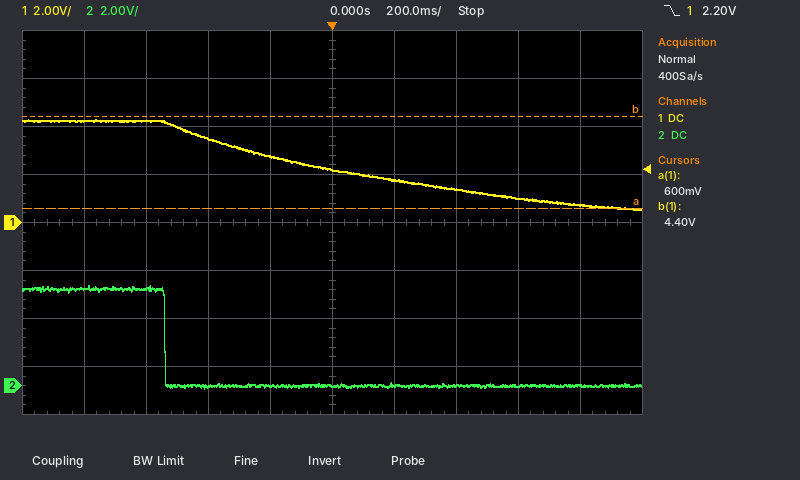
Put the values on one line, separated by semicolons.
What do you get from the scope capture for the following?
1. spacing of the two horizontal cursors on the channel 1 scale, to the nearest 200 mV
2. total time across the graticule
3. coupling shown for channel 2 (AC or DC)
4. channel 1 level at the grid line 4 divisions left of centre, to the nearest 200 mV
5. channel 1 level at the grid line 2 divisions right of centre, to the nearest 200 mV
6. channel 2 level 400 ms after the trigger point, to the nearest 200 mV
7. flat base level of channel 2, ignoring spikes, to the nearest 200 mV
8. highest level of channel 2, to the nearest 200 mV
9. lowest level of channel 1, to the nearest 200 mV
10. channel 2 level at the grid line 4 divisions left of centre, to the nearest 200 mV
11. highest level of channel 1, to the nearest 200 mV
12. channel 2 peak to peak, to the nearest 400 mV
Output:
3.8 V; 2 s; DC; 4.2 V; 1.4 V; 0.0 V; 0.0 V; 4.2 V; 600 mV; 4.0 V; 4.2 V; 4.4 V
